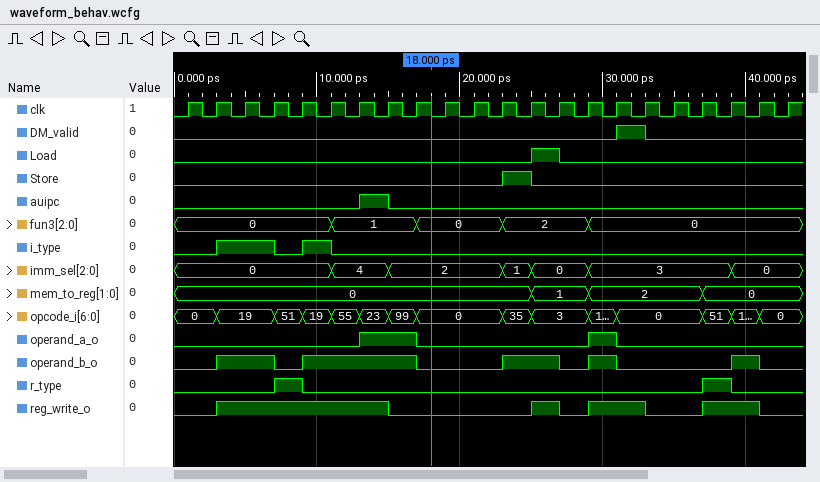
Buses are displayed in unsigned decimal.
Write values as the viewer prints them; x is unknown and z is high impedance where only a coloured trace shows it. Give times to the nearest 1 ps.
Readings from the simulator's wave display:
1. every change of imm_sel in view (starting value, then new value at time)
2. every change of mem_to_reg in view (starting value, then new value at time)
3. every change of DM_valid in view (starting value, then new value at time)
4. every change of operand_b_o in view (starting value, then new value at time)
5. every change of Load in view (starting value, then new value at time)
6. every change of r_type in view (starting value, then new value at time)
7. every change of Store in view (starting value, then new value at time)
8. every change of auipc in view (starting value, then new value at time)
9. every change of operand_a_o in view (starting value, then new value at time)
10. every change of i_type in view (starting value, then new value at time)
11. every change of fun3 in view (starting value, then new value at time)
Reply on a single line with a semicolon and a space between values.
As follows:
0, 4 at 11 ps, 2 at 15 ps, 1 at 23 ps, 0 at 25 ps, 3 at 29 ps, 0 at 39 ps; 0, 1 at 25 ps, 2 at 29 ps, 0 at 37 ps; 0, 1 at 31 ps, 0 at 33 ps; 0, 1 at 3 ps, 0 at 7 ps, 1 at 9 ps, 0 at 17 ps, 1 at 23 ps, 0 at 27 ps, 1 at 29 ps, 0 at 31 ps, 1 at 39 ps, 0 at 41 ps; 0, 1 at 25 ps, 0 at 27 ps; 0, 1 at 7 ps, 0 at 9 ps, 1 at 37 ps, 0 at 39 ps; 0, 1 at 23 ps, 0 at 25 ps; 0, 1 at 13 ps, 0 at 15 ps; 0, 1 at 13 ps, 0 at 17 ps, 1 at 29 ps, 0 at 31 ps; 0, 1 at 3 ps, 0 at 7 ps, 1 at 9 ps, 0 at 11 ps; 0, 1 at 11 ps, 0 at 17 ps, 2 at 23 ps, 0 at 29 ps
